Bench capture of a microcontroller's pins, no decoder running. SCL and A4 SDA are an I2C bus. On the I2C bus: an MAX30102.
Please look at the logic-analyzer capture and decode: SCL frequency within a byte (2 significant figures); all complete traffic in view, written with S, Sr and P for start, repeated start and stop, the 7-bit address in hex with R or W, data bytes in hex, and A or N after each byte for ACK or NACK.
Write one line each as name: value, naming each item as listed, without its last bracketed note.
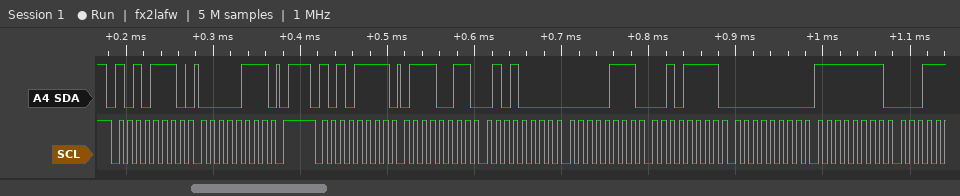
SCL frequency within a byte: 100 kHz
all complete traffic in view, written with S, Sr and P for start, repeated start and stop, the 7-bit address in hex with R or W, data bytes in hex, and A or N after each byte for ACK or NACK: S 57W A 07 A P S 57R A 73 A 50 A 07 A 2F A 00 A FF A
